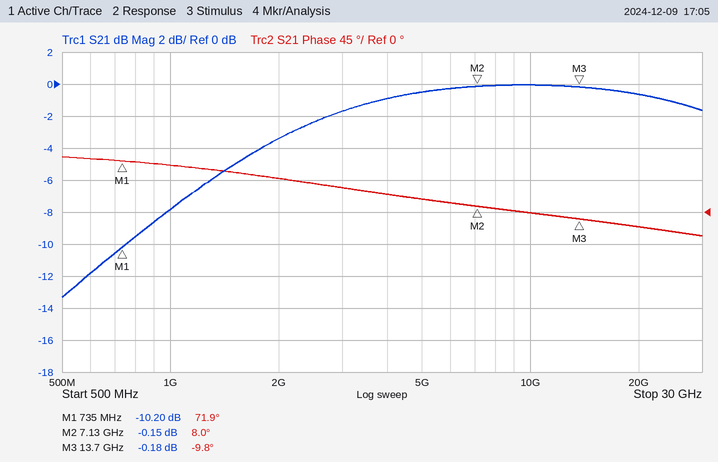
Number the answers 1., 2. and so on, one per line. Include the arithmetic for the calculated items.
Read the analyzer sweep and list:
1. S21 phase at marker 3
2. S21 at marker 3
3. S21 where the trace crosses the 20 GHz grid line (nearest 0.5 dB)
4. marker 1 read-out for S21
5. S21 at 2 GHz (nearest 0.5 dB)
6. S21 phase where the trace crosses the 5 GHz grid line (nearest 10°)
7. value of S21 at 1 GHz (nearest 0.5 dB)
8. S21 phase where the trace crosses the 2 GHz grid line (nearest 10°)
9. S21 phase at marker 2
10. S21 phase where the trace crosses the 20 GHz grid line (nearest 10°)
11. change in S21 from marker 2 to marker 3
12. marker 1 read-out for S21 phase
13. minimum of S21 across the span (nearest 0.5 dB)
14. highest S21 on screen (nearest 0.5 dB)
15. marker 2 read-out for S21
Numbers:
1. -9.8°
2. -0.18 dB
3. -0.5 dB
4. -10.20 dB
5. -3.5 dB
6. 20°
7. -8.0 dB
8. 50°
9. 8.0°
10. -20°
11. -0.18 − (-0.15) = -0.03 dB
12. 71.9°
13. -13.5 dB
14. 0.0 dB
15. -0.15 dB
